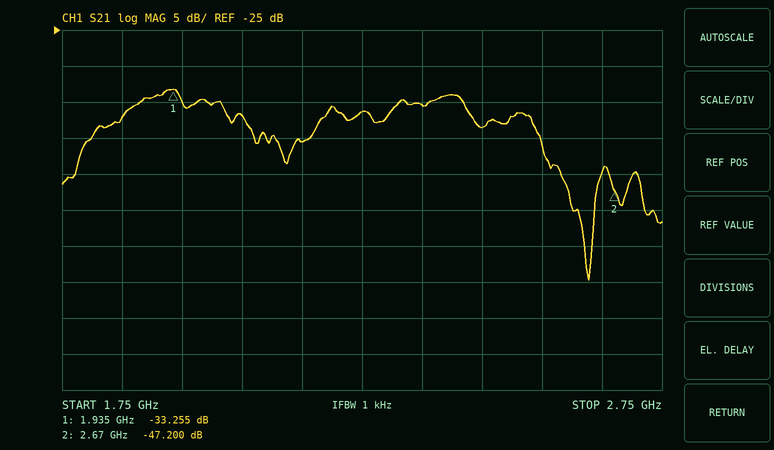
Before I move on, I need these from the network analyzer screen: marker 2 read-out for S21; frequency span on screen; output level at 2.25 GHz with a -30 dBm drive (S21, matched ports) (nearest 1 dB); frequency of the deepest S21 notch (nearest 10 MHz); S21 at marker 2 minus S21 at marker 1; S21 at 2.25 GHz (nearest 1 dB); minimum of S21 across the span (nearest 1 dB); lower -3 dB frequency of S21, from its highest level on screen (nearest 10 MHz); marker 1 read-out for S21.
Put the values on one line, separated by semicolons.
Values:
-47.200 dB; 1 GHz; -66 dBm; 2.63 GHz; -13.945 dB; -36 dB; -60 dB; 1.86 GHz; -33.255 dB
